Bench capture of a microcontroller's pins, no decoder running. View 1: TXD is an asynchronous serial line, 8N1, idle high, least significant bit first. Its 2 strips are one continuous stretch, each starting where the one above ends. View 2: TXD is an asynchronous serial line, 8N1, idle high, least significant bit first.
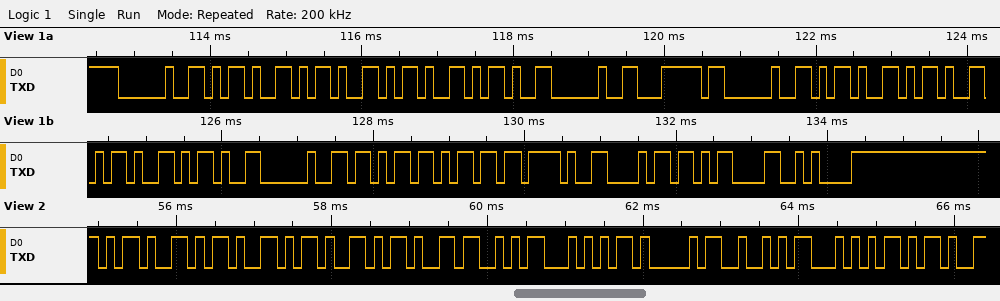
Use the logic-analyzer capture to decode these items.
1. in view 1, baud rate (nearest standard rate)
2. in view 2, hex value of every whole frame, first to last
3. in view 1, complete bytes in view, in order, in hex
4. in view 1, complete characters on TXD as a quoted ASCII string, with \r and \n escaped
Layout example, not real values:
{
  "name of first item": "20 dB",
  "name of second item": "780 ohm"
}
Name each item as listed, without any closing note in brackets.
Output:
{
  "in view 1, baud rate": "9600 baud",
  "in view 2, hex value of every whole frame, first to last": "0x2D 0x2D 0x2D 0x2D 0x53 0x54 0x41 0x52 0x54 0x2D",
  "in view 1, complete bytes in view, in order, in hex": "20 2D 2D 2D 2D 20 7C 20 2D 2D 2D 2D 20 6B 6D 2F 68 0D 0A",
  "in view 1, complete characters on TXD as a quoted ASCII string, with \\r and \\n escaped": "\" ---- | ---- km/h\\r\\n\""
}
